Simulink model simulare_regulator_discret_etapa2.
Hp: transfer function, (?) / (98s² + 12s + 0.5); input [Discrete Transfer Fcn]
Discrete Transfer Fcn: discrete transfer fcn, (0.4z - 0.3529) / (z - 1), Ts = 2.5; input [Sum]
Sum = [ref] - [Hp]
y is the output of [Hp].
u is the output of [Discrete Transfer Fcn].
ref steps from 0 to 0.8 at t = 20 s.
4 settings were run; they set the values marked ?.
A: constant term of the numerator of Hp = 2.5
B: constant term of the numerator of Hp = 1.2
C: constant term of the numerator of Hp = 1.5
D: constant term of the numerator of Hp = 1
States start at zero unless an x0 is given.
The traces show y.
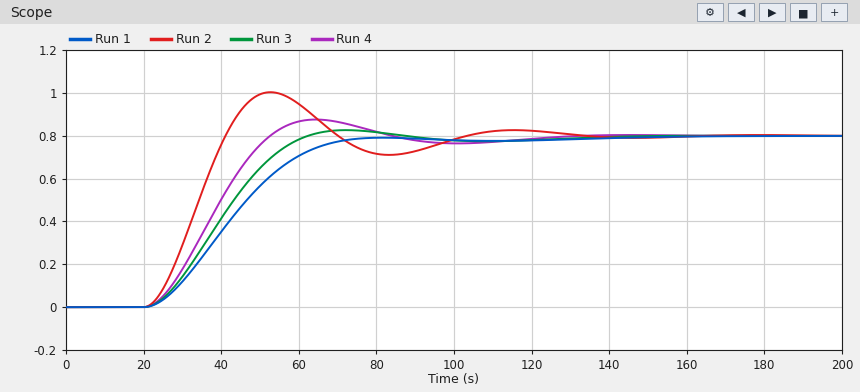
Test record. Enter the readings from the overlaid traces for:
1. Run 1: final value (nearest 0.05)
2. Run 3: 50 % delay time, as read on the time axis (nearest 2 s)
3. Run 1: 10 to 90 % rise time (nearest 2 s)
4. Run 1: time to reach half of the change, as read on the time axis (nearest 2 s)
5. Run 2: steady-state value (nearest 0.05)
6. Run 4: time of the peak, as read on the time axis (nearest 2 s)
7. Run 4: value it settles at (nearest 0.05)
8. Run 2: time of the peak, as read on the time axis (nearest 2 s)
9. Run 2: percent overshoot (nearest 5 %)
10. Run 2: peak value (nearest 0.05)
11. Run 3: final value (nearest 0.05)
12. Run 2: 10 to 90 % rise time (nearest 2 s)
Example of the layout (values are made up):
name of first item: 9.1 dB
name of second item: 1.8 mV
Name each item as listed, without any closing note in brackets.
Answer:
Run 1: final value: 0.80
Run 3: 50 % delay time, as read on the time axis: 40 s
Run 1: 10 to 90 % rise time: 34 s
Run 1: time to reach half of the change, as read on the time axis: 42 s
Run 2: steady-state value: 0.80
Run 4: time of the peak, as read on the time axis: 64 s
Run 4: value it settles at: 0.80
Run 2: time of the peak, as read on the time axis: 52 s
Run 2: percent overshoot: 25 %
Run 2: peak value: 1.00
Run 3: final value: 0.80
Run 2: 10 to 90 % rise time: 14 s
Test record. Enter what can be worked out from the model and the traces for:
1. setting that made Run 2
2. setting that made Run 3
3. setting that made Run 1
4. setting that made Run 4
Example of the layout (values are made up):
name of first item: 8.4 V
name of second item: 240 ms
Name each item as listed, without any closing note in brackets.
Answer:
setting that made Run 2: A
setting that made Run 3: B
setting that made Run 1: D
setting that made Run 4: C
